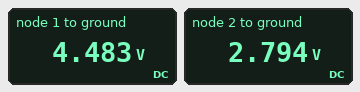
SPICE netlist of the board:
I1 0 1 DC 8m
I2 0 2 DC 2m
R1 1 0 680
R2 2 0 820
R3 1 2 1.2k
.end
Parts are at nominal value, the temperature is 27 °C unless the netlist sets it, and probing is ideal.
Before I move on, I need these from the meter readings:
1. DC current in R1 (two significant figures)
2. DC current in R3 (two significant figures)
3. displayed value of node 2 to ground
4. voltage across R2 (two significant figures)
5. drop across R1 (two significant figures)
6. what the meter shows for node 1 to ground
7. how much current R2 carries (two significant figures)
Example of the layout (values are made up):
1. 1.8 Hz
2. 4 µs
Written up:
1. 6.6 mA
2. 1.4 mA
3. 2.794 V
4. 2.8 V
5. 4.5 V
6. 4.483 V
7. 3.4 mA
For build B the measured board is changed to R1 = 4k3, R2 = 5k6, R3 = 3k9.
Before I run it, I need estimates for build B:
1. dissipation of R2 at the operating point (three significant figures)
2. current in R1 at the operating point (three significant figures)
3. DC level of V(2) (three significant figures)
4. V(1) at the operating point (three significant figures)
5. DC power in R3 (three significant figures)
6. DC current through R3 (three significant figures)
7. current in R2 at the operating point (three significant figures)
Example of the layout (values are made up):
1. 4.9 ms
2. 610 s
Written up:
1. 75.9 mW
2. 6.32 mA
3. 20.6 V
4. 27.2 V
5. 11.0 mW
6. 1.68 mA
7. 3.68 mA
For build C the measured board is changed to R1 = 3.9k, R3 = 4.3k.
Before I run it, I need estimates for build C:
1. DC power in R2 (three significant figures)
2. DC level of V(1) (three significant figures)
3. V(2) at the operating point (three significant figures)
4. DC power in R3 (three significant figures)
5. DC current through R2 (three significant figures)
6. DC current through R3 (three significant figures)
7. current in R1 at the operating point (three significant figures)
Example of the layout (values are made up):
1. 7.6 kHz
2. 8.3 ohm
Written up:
1. 22.8 mW
2. 18.4 V
3. 4.33 V
4. 46.2 mW
5. 5.28 mA
6. 3.28 mA
7. 4.72 mA
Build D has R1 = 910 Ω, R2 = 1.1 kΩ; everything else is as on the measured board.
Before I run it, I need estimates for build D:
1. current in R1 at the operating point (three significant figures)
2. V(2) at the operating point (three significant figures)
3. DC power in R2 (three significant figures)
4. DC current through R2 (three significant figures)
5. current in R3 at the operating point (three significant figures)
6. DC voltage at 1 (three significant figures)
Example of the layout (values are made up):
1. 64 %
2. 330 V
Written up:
1. 6.42 mA
2. 3.94 V
3. 14.1 mW
4. 3.58 mA
5. 1.58 mA
6. 5.84 V
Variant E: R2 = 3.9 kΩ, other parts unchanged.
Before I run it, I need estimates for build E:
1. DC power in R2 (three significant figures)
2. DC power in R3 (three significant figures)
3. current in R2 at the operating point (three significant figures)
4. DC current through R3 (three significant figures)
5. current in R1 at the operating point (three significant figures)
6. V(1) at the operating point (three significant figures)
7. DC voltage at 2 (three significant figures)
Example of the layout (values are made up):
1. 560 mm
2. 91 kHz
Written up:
1. 9.88 mW
2. 200 µW
3. 1.59 mA
4. 408 µA
5. 8.41 mA
6. 5.72 V
7. 6.21 V
